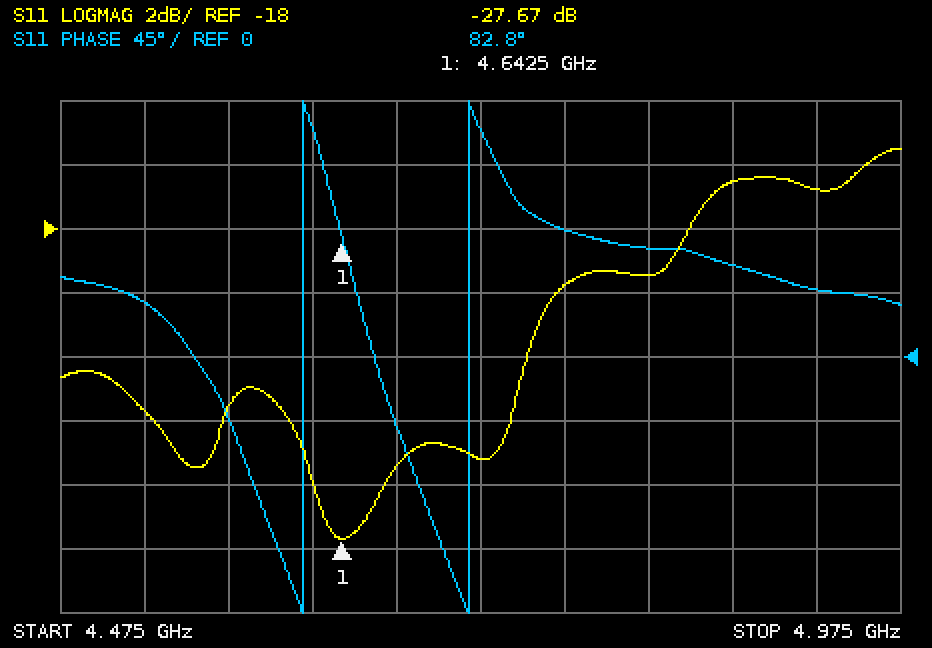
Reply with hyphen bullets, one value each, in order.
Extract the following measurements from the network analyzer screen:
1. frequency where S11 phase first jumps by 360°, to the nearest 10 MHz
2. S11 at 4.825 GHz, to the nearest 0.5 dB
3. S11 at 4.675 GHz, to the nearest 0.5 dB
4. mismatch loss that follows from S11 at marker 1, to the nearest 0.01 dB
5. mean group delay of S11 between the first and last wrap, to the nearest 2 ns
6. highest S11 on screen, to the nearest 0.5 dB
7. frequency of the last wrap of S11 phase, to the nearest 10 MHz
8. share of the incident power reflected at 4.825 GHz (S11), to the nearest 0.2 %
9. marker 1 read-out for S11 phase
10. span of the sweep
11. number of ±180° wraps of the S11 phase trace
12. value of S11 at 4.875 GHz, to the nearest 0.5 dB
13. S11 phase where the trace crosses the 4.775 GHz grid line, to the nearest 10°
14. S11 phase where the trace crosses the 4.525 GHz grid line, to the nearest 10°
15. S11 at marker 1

- 4.62 GHz
- -19.5 dB
- -25.5 dB
- 0.01 dB
- 10 ns
- -15.5 dB
- 4.72 GHz
- 1.2 %
- 82.8°
- 500 MHz
- 2
- -16.5 dB
- 90°
- 40°
- -27.67 dB
